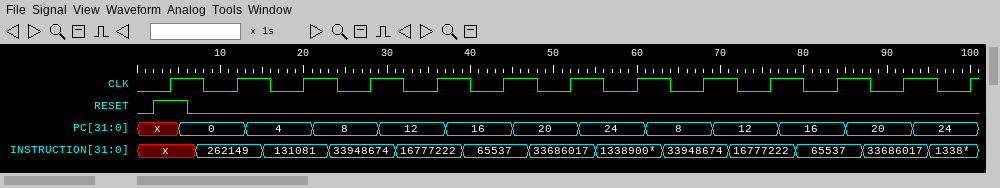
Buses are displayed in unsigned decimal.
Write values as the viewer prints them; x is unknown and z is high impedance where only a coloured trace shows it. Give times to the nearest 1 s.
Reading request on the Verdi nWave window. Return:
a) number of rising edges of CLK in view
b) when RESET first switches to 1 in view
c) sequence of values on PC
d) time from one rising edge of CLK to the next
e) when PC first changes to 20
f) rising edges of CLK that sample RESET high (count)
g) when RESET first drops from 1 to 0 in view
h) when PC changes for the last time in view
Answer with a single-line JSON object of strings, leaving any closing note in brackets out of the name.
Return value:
{"number of rising edges of CLK in view": "13", "when RESET first switches to 1 in view": "2 s", "sequence of values on PC": "x, 0, 4, 8, 12, 16, 20, 24, 8, 12, 16, 20, 24", "time from one rising edge of CLK to the next": "8 s", "when PC first changes to 20": "45 s", "rising edges of CLK that sample RESET high": "1", "when RESET first drops from 1 to 0 in view": "6 s", "when PC changes for the last time in view": "93 s"}
